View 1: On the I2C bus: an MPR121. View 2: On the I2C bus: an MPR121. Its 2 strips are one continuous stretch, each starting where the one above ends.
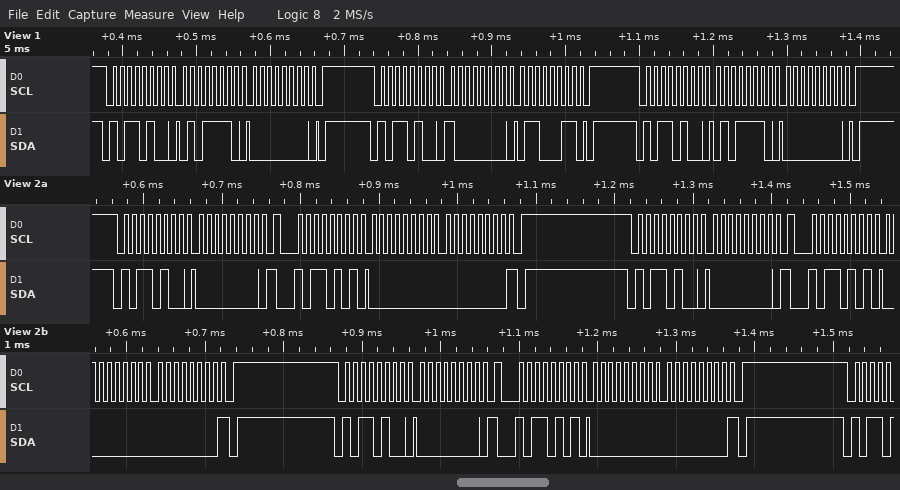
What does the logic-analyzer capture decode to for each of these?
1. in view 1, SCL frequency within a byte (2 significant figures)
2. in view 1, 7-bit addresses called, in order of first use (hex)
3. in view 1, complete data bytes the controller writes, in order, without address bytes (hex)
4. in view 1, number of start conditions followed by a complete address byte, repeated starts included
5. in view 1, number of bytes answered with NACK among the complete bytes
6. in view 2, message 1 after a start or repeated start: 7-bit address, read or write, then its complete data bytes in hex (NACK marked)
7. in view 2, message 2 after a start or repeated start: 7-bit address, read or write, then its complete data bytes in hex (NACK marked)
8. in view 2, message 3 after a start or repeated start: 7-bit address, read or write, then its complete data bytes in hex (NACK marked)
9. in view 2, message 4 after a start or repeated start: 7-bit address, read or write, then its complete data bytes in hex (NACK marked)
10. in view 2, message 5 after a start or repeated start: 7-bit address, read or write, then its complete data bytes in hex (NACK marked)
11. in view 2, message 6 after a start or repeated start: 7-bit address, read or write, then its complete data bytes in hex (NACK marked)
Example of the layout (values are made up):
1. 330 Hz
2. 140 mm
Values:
1. 100 kHz
2. 0x5A
3. 5E 00 80 63 5E 00
4. 3
5. 0
6. 0x5A write: 00
7. 0x5A read: 00 00 NACK
8. 0x5A write: 00
9. 0x5A read: 00 00 NACK
10. 0x5A write: 00
11. 0x5A read: 00 00 NACK
